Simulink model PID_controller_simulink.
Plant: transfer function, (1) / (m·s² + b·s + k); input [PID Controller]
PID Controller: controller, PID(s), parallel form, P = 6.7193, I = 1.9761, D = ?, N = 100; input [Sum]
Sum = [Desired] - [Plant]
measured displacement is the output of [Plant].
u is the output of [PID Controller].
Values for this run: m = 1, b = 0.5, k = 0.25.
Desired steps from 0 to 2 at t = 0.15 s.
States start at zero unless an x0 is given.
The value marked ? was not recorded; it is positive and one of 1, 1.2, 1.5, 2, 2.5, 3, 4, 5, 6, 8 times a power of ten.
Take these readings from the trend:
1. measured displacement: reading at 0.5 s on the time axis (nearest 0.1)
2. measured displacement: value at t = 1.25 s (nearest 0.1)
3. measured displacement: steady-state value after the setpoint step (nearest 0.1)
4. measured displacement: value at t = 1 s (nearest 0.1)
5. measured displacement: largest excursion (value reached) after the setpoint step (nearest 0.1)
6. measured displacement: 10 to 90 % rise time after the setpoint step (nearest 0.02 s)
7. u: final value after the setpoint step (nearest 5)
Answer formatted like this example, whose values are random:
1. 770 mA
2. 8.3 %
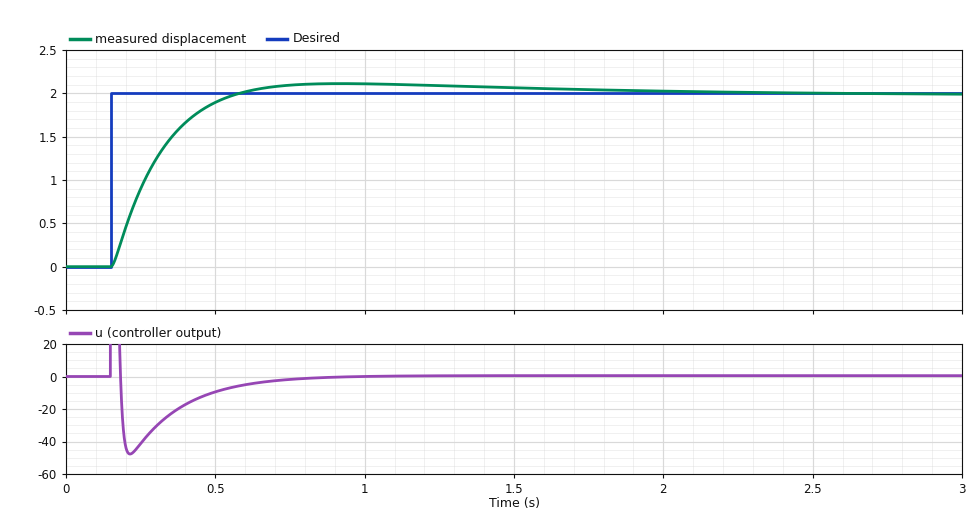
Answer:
1. 1.9
2. 2.1
3. 2.0
4. 2.1
5. 2.1
6. 0.28 s
7. 0
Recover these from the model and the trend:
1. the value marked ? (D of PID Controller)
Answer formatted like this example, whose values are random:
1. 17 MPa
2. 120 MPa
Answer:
1. 6
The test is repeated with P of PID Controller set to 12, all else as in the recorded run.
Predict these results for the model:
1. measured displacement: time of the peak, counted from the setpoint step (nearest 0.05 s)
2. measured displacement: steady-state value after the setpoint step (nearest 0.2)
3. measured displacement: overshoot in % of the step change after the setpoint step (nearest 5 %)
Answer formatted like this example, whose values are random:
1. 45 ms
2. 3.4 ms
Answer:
1. 0.60 s
2. 2.0
3. 10 %
